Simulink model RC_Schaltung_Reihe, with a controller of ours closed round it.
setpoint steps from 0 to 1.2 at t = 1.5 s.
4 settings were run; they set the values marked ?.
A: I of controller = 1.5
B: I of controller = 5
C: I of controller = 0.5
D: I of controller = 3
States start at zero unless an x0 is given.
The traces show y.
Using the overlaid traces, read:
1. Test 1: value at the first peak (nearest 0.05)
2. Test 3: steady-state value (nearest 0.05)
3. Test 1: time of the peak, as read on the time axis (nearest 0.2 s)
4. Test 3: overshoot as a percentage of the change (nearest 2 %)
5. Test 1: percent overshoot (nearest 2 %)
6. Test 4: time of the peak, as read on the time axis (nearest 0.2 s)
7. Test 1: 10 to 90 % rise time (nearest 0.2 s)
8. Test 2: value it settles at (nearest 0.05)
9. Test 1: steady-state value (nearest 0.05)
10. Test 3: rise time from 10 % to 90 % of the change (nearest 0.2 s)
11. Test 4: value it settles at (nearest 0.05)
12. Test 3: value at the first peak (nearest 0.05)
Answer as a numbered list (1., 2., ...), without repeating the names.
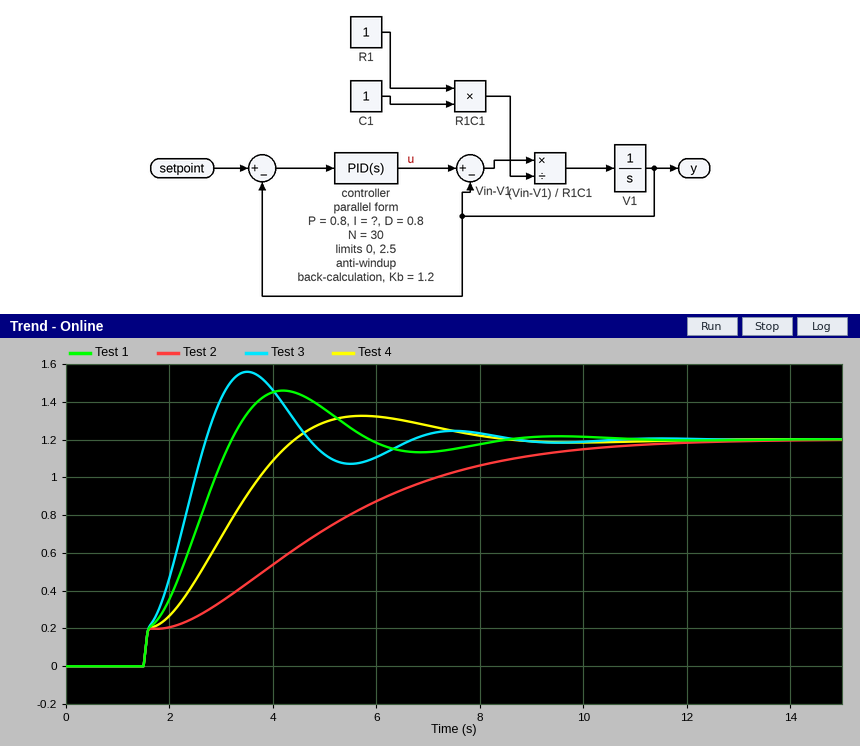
1. 1.45
2. 1.20
3. 4.2 s
4. 30 %
5. 22 %
6. 5.8 s
7. 1.4 s
8. 1.20
9. 1.20
10. 1.0 s
11. 1.20
12. 1.55
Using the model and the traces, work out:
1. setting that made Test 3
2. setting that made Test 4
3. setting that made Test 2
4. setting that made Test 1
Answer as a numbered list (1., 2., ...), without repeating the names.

1. B
2. A
3. C
4. D
